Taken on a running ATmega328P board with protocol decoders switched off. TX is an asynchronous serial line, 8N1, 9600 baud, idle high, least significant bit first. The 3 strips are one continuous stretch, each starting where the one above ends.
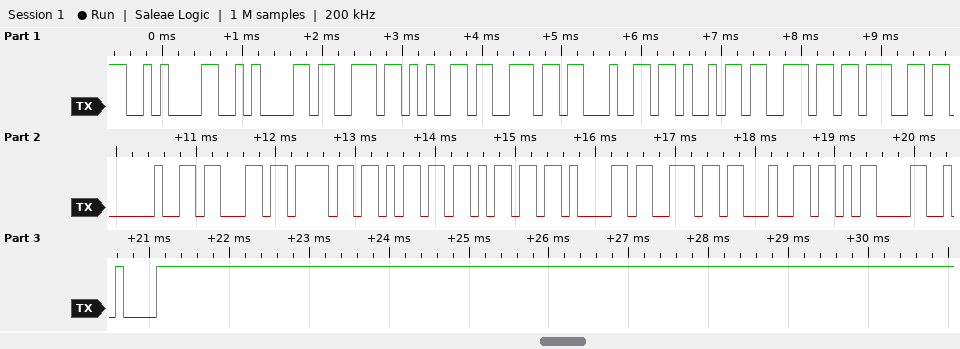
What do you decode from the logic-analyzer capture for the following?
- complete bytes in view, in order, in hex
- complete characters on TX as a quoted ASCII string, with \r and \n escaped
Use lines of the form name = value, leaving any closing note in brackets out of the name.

complete bytes in view, in order, in hex = 0A 0A 73 65 6E 64 69 6E 67 20 63 6F 6D 6D 61 6E 64 0D 0A
complete characters on TX as a quoted ASCII string, with \r and \n escaped = "\n\nsending command\r\n"
